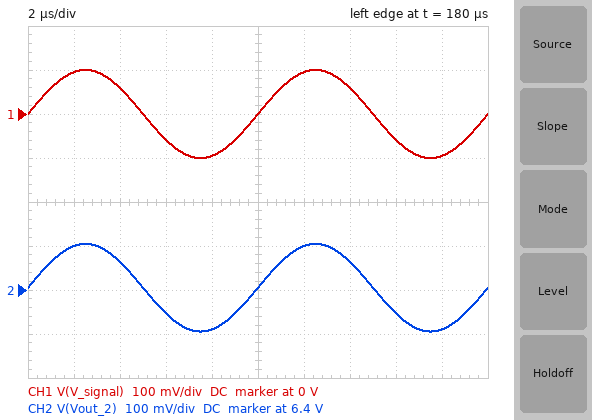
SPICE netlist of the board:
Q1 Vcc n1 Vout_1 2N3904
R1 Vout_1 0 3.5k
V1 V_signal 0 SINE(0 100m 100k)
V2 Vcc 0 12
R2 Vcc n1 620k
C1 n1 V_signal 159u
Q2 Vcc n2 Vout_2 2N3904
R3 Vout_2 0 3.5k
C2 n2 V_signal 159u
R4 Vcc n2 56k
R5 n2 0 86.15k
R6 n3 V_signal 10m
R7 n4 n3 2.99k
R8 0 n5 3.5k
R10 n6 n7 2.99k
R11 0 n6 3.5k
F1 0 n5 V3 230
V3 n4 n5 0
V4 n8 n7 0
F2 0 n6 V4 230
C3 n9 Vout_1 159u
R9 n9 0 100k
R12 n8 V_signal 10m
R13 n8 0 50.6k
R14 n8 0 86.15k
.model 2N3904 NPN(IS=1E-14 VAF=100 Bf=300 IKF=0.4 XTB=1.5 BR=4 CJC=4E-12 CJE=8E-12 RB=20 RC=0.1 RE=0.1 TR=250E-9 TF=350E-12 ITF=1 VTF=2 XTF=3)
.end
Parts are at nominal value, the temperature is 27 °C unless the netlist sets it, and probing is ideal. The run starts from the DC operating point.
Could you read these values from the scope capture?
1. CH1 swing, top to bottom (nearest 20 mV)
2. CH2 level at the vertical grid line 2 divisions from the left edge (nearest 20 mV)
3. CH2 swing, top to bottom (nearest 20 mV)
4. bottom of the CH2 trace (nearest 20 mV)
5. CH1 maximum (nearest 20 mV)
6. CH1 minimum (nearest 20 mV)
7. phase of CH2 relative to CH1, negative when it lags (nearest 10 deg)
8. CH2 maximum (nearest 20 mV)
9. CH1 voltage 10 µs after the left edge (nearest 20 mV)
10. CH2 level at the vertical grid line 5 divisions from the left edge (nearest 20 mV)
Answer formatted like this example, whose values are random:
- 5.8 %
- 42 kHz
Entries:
- 200 mV
- 6.46 V
- 200 mV
- 6.30 V
- 100 mV
- -100 mV
- 0 deg
- 6.50 V
- 0 V
- 6.40 V
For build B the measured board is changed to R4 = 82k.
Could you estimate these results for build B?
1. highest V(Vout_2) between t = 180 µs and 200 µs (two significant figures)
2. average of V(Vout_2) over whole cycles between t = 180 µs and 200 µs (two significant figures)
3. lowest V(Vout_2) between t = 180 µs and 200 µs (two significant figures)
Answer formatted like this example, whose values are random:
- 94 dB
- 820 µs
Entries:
- 5.4 V
- 5.3 V
- 5.2 V
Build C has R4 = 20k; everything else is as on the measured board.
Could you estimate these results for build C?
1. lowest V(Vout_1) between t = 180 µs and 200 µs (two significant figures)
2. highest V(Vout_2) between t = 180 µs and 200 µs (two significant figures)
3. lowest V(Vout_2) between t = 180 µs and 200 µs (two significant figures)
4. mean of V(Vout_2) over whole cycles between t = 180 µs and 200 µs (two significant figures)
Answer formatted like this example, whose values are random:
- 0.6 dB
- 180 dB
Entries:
- 7.1 V
- 9.0 V
- 8.8 V
- 8.9 V
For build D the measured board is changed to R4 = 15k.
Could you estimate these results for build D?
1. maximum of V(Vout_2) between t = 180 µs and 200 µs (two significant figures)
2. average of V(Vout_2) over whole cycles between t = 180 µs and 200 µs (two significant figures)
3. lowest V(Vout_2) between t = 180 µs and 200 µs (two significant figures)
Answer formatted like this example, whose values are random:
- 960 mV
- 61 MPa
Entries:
- 9.5 V
- 9.4 V
- 9.3 V
